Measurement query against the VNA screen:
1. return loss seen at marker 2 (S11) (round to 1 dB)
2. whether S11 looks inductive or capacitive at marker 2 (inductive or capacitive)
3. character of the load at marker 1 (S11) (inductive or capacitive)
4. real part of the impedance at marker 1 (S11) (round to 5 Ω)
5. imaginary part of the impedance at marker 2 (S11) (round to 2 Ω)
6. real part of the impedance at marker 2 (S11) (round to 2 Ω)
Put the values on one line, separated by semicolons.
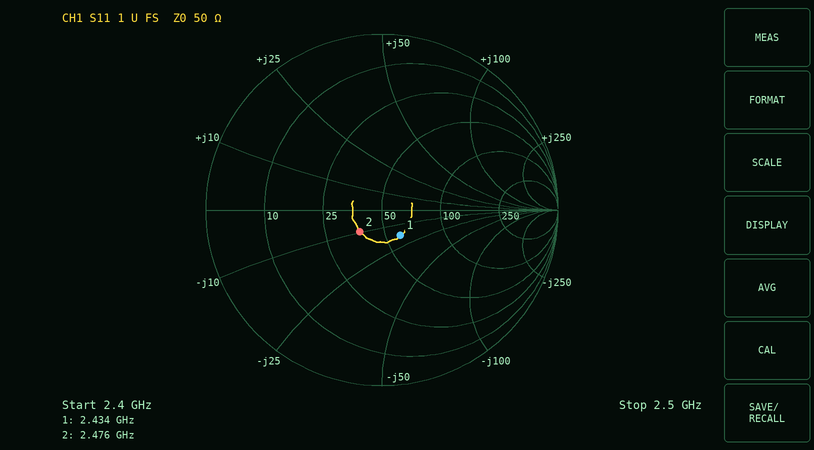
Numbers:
15 dB; capacitive; capacitive; 60 Ω; -10 Ω; 38 Ω
